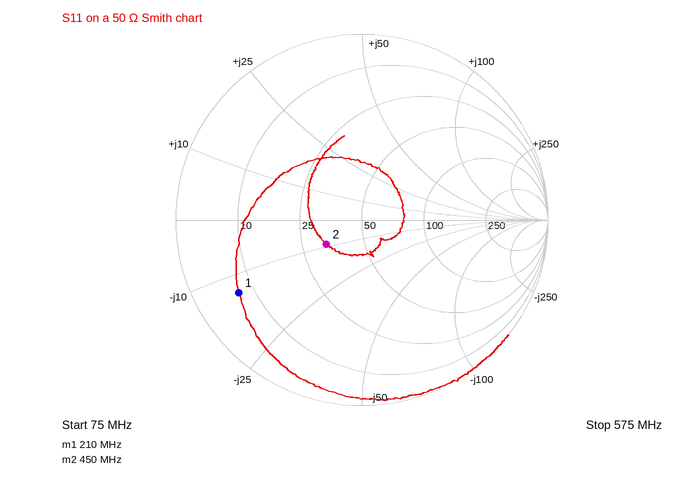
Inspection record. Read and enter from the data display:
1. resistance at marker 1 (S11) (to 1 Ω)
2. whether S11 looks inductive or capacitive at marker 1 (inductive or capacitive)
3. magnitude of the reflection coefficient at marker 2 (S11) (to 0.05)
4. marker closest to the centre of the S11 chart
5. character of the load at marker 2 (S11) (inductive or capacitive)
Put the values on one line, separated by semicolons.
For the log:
7 Ω; capacitive; 0.25; marker 2; capacitive
